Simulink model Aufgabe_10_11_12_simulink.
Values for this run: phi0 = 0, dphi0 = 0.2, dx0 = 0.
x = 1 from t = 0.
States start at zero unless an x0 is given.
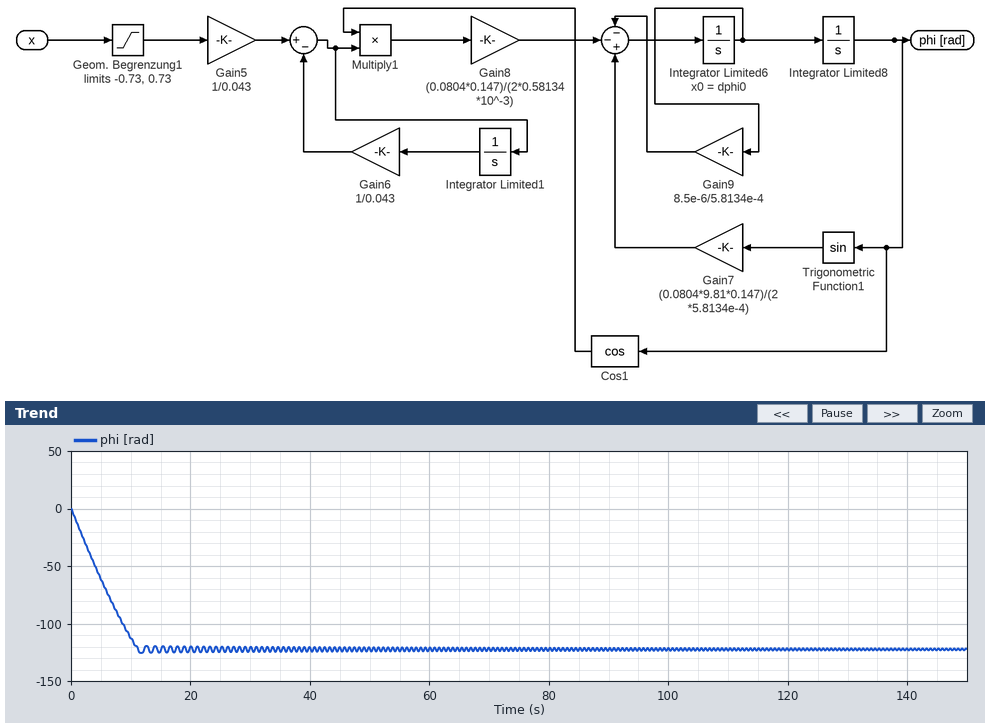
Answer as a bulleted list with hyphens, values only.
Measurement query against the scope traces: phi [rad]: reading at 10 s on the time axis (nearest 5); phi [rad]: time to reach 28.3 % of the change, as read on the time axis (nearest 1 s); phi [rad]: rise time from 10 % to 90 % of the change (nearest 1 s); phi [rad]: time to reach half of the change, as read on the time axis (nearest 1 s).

- -115
- 3 s
- 9 s
- 5 s
